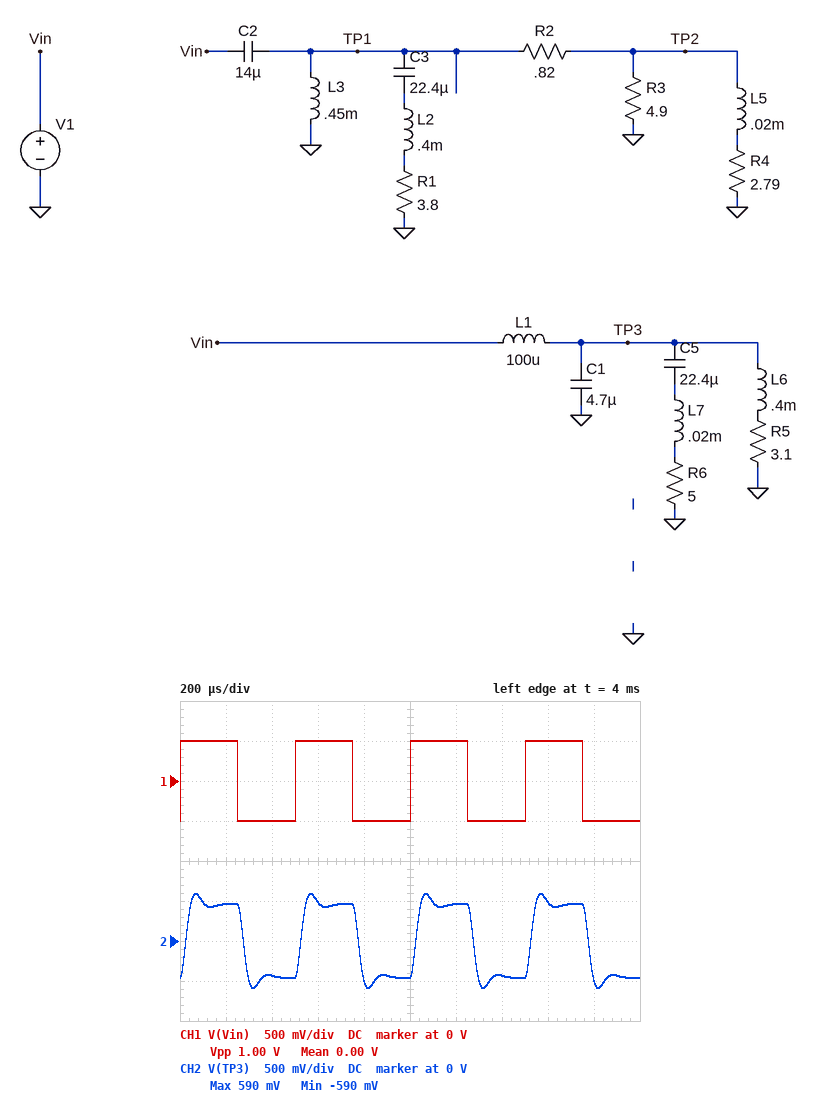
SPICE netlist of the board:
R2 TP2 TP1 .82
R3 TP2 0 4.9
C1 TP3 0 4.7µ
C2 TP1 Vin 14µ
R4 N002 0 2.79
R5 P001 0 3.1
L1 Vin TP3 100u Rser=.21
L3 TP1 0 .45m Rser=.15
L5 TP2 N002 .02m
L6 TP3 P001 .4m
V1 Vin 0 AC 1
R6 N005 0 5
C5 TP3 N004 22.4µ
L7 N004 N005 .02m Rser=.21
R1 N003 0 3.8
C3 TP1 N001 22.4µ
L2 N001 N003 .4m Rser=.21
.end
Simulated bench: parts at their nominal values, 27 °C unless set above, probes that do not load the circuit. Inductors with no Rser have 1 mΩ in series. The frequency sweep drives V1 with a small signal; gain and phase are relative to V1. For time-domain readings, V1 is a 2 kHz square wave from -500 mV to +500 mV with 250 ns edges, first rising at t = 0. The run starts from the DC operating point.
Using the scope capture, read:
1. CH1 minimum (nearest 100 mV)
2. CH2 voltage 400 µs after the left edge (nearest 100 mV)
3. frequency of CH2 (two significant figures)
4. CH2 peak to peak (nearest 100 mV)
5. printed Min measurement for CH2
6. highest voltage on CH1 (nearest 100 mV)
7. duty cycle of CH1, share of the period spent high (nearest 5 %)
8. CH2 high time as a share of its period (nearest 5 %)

-500 mV
-400 mV
2.0 kHz
1.2 V
-590 mV
500 mV
50 %
50 %
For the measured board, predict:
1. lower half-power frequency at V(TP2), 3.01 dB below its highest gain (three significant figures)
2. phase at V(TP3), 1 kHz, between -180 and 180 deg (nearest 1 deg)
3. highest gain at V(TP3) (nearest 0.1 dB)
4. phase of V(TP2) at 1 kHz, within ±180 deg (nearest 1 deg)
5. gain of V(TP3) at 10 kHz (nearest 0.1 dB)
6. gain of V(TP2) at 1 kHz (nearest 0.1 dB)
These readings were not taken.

4.65 kHz
-8 deg
0.3 dB
107 deg
-2.6 dB
-18.9 dB
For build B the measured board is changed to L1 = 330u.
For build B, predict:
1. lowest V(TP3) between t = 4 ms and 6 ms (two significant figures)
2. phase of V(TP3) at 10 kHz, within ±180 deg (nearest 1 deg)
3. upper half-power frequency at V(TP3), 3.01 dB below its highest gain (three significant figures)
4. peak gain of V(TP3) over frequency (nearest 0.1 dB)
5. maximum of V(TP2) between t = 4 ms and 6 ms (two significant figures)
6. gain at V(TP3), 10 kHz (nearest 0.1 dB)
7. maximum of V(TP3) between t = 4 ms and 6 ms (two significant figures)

-410 mV
-133 deg
2.72 kHz
-0.6 dB
840 mV
-15.0 dB
410 mV
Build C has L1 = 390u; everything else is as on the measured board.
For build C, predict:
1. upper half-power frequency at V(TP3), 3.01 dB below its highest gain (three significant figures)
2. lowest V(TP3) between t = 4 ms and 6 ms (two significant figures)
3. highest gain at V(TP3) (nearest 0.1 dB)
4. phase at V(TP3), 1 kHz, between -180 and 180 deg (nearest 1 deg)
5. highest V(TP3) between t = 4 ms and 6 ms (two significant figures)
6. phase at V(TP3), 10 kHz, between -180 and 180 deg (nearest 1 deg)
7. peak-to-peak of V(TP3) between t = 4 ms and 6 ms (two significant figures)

1.96 kHz
-390 mV
-0.6 dB
-29 deg
390 mV
-135 deg
780 mV
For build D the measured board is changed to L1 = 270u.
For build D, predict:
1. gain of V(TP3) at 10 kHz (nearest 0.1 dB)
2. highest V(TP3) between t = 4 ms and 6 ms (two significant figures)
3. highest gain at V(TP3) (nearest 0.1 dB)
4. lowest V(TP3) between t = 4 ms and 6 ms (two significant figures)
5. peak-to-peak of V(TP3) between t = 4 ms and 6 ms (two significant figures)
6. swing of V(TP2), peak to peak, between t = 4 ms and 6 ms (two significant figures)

-13.0 dB
420 mV
-0.6 dB
-420 mV
840 mV
1.7 V
